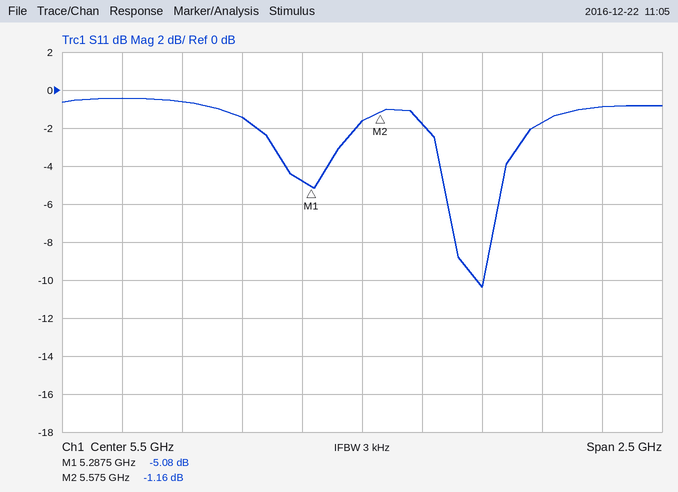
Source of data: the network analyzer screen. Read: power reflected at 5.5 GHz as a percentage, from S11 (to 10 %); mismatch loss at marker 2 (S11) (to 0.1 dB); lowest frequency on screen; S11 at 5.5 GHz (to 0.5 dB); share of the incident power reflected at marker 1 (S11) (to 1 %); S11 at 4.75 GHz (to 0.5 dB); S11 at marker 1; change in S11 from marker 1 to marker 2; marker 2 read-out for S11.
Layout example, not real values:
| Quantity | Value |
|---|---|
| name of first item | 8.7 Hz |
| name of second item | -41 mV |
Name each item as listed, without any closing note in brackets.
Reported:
| Quantity | Value |
|---|---|
| power reflected at 5.5 GHz as a percentage, from S11 | 70 % |
| mismatch loss at marker 2 (S11) | 6.3 dB |
| lowest frequency on screen | 4.25 GHz |
| S11 at 5.5 GHz | -1.5 dB |
| share of the incident power reflected at marker 1 (S11) | 31 % |
| S11 at 4.75 GHz | -0.5 dB |
| S11 at marker 1 | -5.08 dB |
| change in S11 from marker 1 to marker 2 | 3.92 dB |
| marker 2 read-out for S11 | -1.16 dB |
